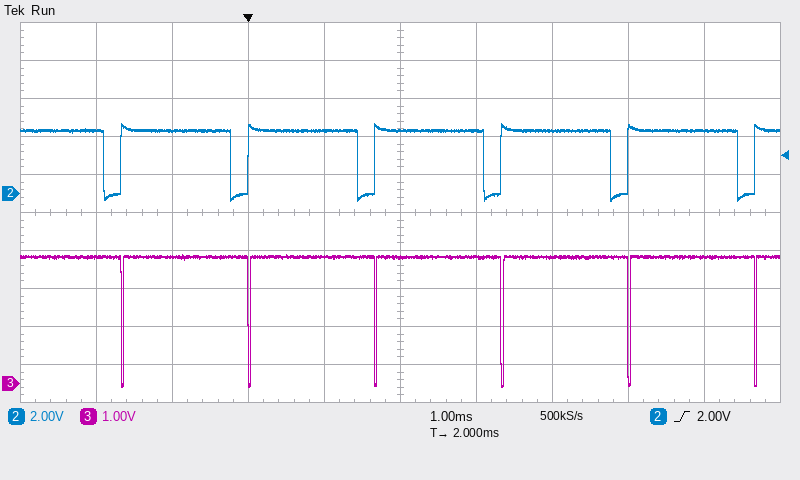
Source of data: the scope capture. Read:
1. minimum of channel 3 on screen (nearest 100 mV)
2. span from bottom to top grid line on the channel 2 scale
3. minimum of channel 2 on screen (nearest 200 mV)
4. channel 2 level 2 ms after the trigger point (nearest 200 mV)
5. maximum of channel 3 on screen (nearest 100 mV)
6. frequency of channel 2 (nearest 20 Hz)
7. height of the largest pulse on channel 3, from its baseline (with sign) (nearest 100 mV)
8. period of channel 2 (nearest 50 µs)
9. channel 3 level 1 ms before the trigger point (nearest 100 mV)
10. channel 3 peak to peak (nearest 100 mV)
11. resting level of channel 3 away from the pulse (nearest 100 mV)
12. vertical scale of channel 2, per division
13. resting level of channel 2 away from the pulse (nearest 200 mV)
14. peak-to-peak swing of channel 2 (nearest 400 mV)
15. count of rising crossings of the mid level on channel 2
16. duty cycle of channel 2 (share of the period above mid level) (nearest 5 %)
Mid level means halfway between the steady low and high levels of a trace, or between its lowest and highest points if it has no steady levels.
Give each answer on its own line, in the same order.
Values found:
-100 mV
20 V
-400 mV
3.4 V
3.4 V
600 Hz
-3.4 V
1.65 ms
3.3 V
3.5 V
3.3 V
2 V
3.4 V
4.0 V
6
85 %
